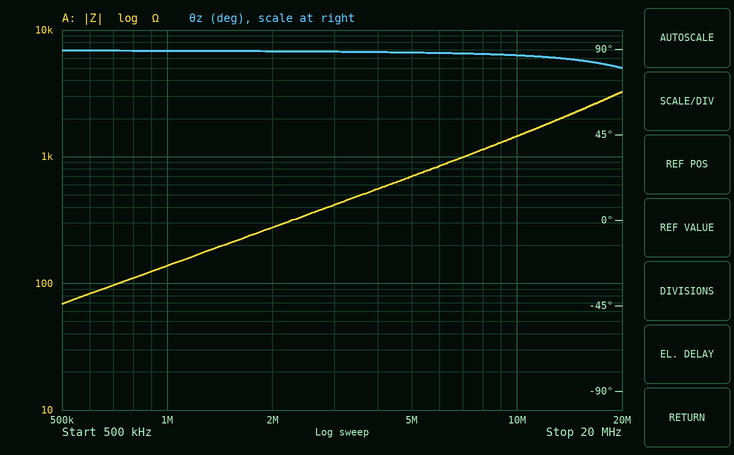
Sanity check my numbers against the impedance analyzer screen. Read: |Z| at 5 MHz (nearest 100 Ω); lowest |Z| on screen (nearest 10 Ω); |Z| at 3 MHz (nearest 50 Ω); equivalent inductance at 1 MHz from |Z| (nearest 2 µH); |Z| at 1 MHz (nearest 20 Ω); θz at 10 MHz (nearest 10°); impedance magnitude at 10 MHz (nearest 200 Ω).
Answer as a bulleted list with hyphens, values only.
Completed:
- 700 Ω
- 70 Ω
- 400 Ω
- 22 µH
- 140 Ω
- 90°
- 1.4 kΩ
